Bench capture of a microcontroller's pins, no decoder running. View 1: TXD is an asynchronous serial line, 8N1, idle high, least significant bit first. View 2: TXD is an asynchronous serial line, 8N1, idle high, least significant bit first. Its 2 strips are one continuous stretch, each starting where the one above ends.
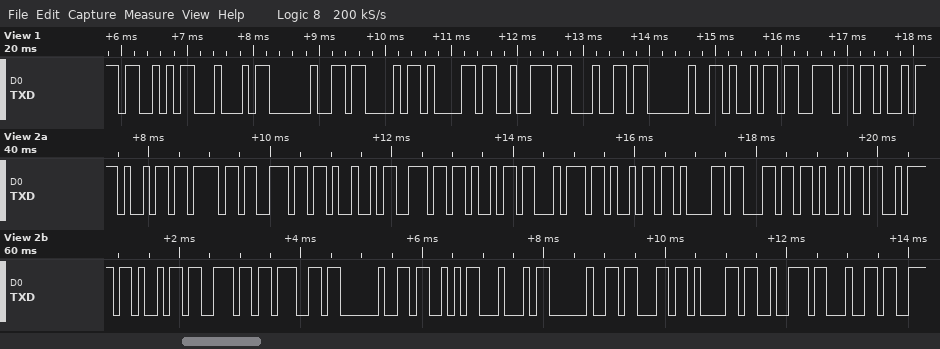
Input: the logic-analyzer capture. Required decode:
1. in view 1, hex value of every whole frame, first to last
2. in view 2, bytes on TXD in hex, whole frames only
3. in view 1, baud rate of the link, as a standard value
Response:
0x53 0x44 0x20 0x43 0x61 0x72 0x64 0x20 0x69 0x6E
69 6F 6E 49 6E 69 74 69 61 6C 69 7A 69 6E 67 20 53 44 20 63 61 72 64
9600 baud
